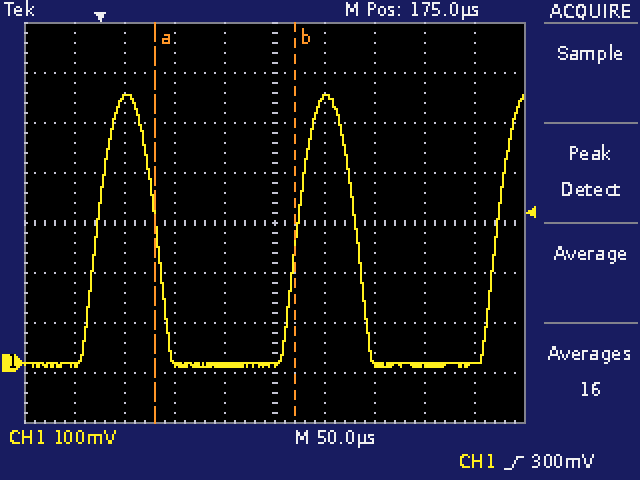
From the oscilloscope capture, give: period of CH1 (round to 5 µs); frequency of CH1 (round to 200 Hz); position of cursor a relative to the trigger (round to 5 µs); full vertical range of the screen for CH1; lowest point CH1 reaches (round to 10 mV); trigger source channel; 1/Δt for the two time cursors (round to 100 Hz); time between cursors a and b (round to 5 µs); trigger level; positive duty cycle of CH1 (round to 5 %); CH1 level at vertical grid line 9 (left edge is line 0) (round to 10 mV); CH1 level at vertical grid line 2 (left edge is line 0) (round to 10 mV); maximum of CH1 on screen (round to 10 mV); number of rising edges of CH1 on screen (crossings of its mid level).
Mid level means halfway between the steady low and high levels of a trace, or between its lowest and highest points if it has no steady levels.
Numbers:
200 µs
5.0 kHz
+55 µs
800 mV
-10 mV
CH1
7.1 kHz
140 µs
300 mV
30 %
0 mV
530 mV
540 mV
3
